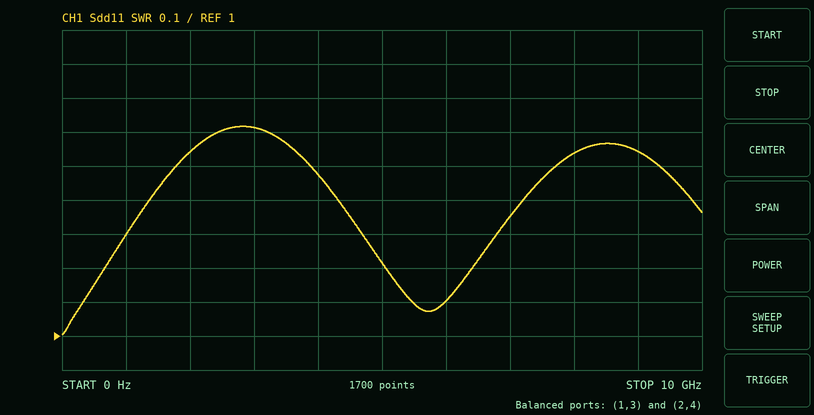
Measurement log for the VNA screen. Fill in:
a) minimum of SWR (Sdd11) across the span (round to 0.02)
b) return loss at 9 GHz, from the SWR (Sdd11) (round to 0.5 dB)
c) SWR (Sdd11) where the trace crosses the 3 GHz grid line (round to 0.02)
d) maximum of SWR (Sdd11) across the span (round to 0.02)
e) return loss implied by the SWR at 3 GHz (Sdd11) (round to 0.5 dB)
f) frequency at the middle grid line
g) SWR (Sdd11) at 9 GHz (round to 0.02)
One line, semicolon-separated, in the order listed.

1.00; 13.5 dB; 1.62; 1.62; 12.5 dB; 5 GHz; 1.54
